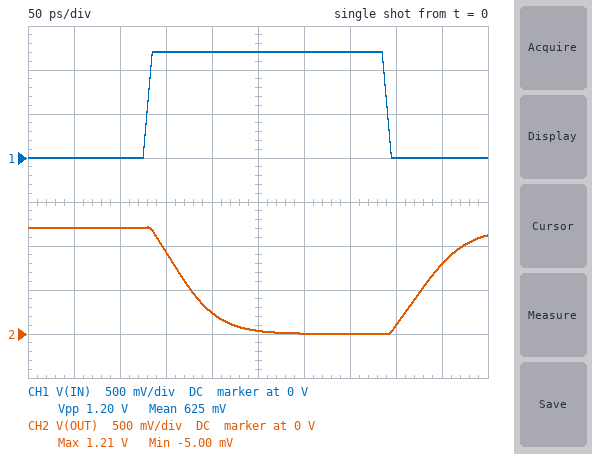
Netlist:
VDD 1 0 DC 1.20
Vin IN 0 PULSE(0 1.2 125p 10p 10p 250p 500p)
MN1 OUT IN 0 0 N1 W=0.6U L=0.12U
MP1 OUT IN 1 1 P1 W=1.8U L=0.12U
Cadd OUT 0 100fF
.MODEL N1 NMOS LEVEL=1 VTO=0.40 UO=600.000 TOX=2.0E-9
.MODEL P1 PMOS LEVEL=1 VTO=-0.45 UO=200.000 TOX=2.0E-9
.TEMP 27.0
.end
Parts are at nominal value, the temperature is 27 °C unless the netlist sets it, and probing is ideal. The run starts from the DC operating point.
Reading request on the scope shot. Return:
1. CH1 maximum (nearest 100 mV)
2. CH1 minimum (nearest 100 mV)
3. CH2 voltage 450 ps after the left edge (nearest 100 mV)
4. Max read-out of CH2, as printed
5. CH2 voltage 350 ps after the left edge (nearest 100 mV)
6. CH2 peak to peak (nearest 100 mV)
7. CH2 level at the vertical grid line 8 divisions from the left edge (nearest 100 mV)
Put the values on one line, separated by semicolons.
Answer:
1.2 V; 0 V; 800 mV; 1.21 V; 0 V; 1.2 V; 100 mV
